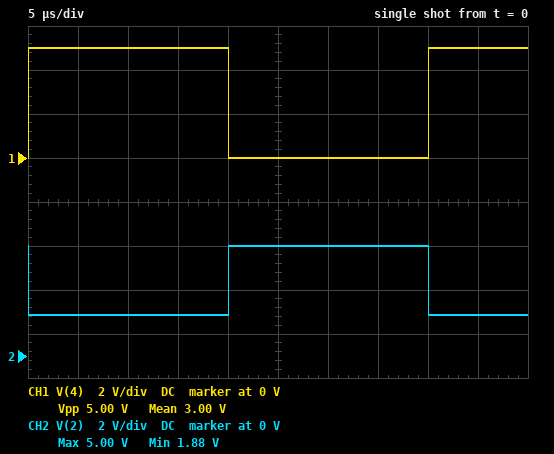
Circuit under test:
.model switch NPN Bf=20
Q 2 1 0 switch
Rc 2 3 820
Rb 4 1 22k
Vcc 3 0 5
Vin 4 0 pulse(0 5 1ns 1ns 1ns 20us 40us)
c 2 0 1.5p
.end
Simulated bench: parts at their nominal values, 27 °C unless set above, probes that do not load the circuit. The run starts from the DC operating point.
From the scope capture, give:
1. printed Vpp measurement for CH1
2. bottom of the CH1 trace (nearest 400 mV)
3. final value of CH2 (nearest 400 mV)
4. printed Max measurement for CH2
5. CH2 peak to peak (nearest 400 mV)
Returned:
5.00 V
0 V
2.0 V
5.00 V
3.2 V
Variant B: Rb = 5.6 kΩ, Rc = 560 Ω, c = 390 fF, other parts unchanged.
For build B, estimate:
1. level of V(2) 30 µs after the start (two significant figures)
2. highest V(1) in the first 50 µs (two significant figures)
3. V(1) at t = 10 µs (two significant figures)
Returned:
5.0 V
840 mV
830 mV
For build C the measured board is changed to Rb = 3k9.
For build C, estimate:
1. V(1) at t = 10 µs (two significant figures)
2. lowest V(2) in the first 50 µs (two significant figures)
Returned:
830 mV
61 mV
